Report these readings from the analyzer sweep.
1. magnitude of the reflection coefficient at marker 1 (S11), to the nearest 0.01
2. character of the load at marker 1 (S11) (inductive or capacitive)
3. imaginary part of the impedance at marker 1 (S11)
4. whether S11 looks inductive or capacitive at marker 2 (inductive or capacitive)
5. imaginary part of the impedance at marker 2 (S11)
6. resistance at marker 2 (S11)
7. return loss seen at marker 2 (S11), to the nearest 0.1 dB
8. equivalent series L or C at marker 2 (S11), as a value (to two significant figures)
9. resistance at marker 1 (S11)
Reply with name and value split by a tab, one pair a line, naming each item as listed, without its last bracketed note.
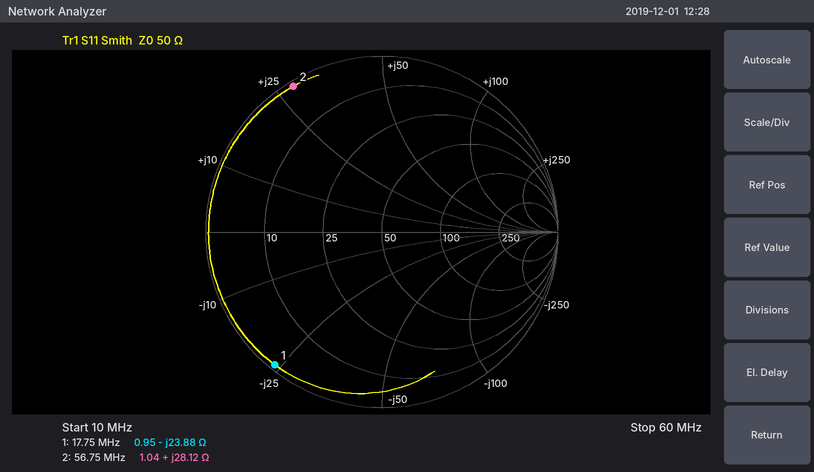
magnitude of the reflection coefficient at marker 1 (S11), to the nearest 0.01	0.97
character of the load at marker 1 (S11)	capacitive
imaginary part of the impedance at marker 1	-23.88 Ω
whether S11 looks inductive or capacitive at marker 2	inductive
imaginary part of the impedance at marker 2	+28.12 Ω
resistance at marker 2	1.04 Ω
return loss seen at marker 2 (S11), to the nearest 0.1 dB	0.3 dB
equivalent series L or C at marker 2 (S11), as a value	79 nH
resistance at marker 1	0.95 Ω
